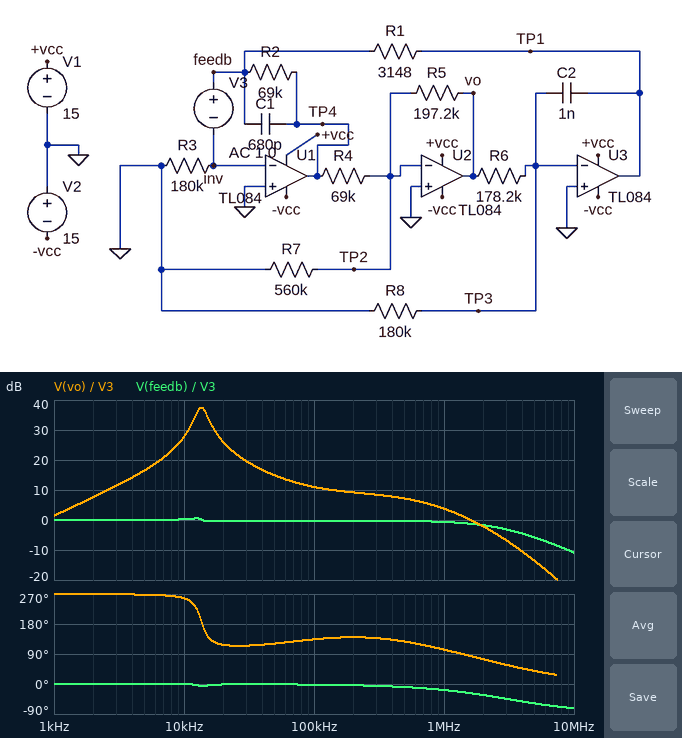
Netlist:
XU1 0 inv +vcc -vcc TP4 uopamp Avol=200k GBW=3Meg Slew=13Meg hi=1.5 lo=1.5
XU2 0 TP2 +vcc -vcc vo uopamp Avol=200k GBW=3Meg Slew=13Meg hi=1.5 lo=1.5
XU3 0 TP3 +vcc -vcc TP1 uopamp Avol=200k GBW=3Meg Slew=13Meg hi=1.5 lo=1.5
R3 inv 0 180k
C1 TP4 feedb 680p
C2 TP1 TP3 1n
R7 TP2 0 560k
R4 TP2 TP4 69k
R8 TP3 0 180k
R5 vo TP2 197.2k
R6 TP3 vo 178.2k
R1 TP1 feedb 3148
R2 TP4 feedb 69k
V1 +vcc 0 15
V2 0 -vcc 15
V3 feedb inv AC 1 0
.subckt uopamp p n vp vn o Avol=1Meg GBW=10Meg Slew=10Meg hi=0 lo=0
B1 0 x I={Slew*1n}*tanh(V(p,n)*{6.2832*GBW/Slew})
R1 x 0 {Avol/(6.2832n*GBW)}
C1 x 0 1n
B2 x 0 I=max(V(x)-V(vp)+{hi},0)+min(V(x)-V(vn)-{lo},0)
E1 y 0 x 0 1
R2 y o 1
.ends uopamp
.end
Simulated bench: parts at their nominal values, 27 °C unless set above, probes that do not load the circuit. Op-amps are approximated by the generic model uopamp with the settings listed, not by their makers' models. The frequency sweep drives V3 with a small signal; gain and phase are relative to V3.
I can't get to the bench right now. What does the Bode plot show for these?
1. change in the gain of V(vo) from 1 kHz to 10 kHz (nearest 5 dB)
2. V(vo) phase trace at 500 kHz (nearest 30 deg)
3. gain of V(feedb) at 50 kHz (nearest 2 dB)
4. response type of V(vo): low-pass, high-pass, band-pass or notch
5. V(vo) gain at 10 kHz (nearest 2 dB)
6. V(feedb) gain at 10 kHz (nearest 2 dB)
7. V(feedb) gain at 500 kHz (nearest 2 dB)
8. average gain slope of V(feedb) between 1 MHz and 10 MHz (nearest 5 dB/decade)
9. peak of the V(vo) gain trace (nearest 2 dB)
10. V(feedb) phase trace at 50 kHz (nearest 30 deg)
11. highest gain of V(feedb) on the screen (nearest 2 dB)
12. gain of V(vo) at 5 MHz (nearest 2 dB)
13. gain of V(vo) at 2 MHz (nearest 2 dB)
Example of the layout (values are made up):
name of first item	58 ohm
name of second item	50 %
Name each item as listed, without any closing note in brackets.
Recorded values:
change in the gain of V(vo) from 1 kHz to 10 kHz	25 dB
V(vo) phase trace at 500 kHz	120 deg
gain of V(feedb) at 50 kHz	0 dB
response type of V(vo): low-pass, high-pass, band-pass or notch	band-pass
V(vo) gain at 10 kHz	28 dB
V(feedb) gain at 10 kHz	0 dB
V(feedb) gain at 500 kHz	0 dB
average gain slope of V(feedb) between 1 MHz and 10 MHz	-10 dB/decade
peak of the V(vo) gain trace	38 dB
V(feedb) phase trace at 50 kHz	0 deg
highest gain of V(feedb) on the screen	0 dB
gain of V(vo) at 5 MHz	-14 dB
gain of V(vo) at 2 MHz	-2 dB
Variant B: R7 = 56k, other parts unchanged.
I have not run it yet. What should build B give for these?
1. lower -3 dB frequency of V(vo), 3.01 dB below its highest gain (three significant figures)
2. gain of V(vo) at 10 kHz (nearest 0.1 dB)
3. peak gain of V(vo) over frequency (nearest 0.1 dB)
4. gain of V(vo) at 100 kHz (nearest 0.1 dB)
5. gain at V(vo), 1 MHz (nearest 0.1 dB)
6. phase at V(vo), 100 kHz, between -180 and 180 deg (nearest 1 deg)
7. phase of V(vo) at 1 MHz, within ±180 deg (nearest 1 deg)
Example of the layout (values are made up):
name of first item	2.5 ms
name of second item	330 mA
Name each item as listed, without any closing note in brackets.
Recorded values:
lower -3 dB frequency of V(vo), 3.01 dB below its highest gain	12.3 kHz
gain of V(vo) at 10 kHz	27.8 dB
peak gain of V(vo) over frequency	38.1 dB
gain of V(vo) at 100 kHz	10.8 dB
gain at V(vo), 1 MHz	0 dB
phase at V(vo), 100 kHz, between -180 and 180 deg	128 deg
phase of V(vo) at 1 MHz, within ±180 deg	90 deg
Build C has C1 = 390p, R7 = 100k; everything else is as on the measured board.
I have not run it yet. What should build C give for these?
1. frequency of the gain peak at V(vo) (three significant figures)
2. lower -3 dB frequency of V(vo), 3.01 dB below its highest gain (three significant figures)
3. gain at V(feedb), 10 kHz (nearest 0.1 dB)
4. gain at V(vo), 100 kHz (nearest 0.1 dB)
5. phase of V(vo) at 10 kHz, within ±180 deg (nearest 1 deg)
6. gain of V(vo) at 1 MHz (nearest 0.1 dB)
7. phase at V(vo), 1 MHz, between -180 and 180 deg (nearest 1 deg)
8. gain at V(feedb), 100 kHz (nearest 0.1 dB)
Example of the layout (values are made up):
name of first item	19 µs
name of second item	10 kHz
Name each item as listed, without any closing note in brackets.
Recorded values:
frequency of the gain peak at V(vo)	17.8 kHz
lower -3 dB frequency of V(vo), 3.01 dB below its highest gain	15.5 kHz
gain at V(feedb), 10 kHz	0.2 dB
gain at V(vo), 100 kHz	13.4 dB
phase of V(vo) at 10 kHz, within ±180 deg	-100 deg
gain of V(vo) at 1 MHz	1.6 dB
phase at V(vo), 1 MHz, between -180 and 180 deg	92 deg
gain at V(feedb), 100 kHz	-0.4 dB
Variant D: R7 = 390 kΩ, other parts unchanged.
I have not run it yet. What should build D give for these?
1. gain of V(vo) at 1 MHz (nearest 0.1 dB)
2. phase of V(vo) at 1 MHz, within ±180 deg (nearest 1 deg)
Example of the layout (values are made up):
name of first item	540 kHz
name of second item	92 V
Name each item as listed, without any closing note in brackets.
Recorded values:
gain of V(vo) at 1 MHz	3.6 dB
phase of V(vo) at 1 MHz, within ±180 deg	102 deg
